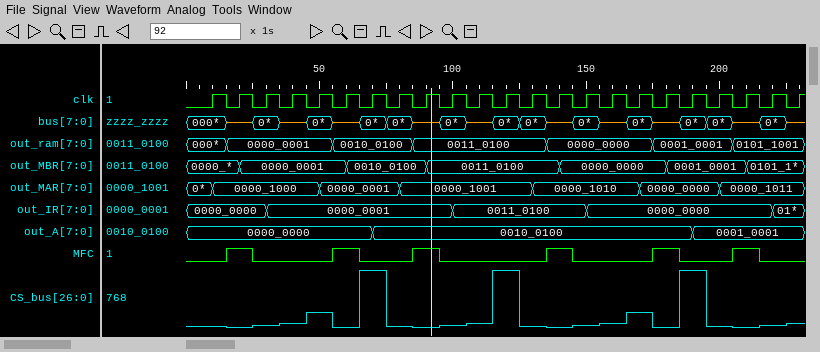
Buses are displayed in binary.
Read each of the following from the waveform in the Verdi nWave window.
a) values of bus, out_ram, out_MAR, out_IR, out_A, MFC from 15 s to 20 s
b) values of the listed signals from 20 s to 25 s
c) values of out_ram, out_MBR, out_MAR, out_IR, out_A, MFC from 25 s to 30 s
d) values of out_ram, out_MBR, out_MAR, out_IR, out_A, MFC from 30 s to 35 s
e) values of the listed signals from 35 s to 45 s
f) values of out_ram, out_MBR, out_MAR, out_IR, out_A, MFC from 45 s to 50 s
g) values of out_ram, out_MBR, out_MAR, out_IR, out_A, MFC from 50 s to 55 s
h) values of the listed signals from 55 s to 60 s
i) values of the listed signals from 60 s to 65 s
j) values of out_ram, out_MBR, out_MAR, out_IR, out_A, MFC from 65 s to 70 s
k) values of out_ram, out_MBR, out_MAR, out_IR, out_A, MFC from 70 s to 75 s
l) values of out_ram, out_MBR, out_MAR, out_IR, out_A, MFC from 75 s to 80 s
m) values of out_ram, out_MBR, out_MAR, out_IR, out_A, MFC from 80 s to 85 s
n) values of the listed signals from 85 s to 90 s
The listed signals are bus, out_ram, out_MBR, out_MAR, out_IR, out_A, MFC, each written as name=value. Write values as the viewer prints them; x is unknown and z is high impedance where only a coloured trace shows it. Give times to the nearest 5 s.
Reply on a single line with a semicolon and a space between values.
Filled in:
bus=z, out_ram=0000_0001, out_MAR=0000_1000, out_IR=0000_0000, out_A=0000_0000, MFC=1; bus=z, out_ram=0000_0001, out_MBR=0000_0001, out_MAR=0000_1000, out_IR=0000_0000, out_A=0000_0000, MFC=1; out_ram=0000_0001, out_MBR=0000_0001, out_MAR=0000_1000, out_IR=0000_0000, out_A=0000_0000, MFC=0; out_ram=0000_0001, out_MBR=0000_0001, out_MAR=0000_1000, out_IR=0000_0001, out_A=0000_0000, MFC=0; bus=z, out_ram=0000_0001, out_MBR=0000_0001, out_MAR=0000_1000, out_IR=0000_0001, out_A=0000_0000, MFC=0; out_ram=0000_0001, out_MBR=0000_0001, out_MAR=0000_1000, out_IR=0000_0001, out_A=0000_0000, MFC=0; out_ram=0000_0001, out_MBR=0000_0001, out_MAR=0000_0001, out_IR=0000_0001, out_A=0000_0000, MFC=0; bus=z, out_ram=0010_0100, out_MBR=0000_0001, out_MAR=0000_0001, out_IR=0000_0001, out_A=0000_0000, MFC=1; bus=z, out_ram=0010_0100, out_MBR=0010_0100, out_MAR=0000_0001, out_IR=0000_0001, out_A=0000_0000, MFC=1; out_ram=0010_0100, out_MBR=0010_0100, out_MAR=0000_0001, out_IR=0000_0001, out_A=0000_0000, MFC=0; out_ram=0010_0100, out_MBR=0010_0100, out_MAR=0000_0001, out_IR=0000_0001, out_A=0010_0100, MFC=0; out_ram=0010_0100, out_MBR=0010_0100, out_MAR=0000_0001, out_IR=0000_0001, out_A=0010_0100, MFC=0; out_ram=0010_0100, out_MBR=0010_0100, out_MAR=0000_1001, out_IR=0000_0001, out_A=0010_0100, MFC=0; bus=z, out_ram=0011_0100, out_MBR=0010_0100, out_MAR=0000_1001, out_IR=0000_0001, out_A=0010_0100, MFC=1
